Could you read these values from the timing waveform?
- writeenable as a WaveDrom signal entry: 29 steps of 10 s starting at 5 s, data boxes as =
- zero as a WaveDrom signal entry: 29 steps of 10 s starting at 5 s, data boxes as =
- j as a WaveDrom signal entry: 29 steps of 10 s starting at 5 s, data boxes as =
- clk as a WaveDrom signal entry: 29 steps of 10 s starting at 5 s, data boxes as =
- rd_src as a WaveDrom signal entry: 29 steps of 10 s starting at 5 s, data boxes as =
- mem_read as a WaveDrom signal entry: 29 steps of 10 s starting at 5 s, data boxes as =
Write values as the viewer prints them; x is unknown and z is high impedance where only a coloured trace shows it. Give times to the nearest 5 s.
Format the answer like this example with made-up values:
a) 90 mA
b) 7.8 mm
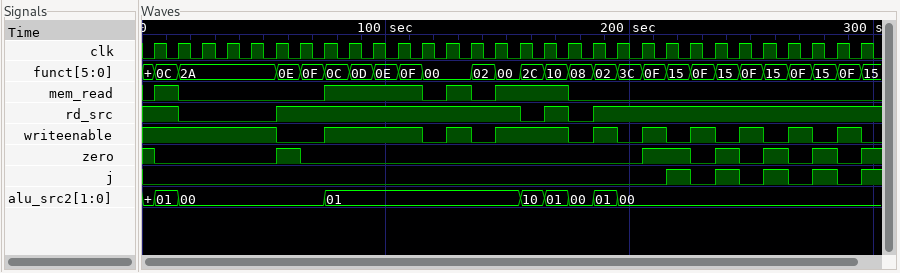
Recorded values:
a) {name: 'writeenable', wave: '1....0.1...0101..010101010101'}
b) {name: 'zero', wave: '0....10.............1.0101010'}
c) {name: 'j', wave: '0....................10101010'}
d) {name: 'clk', wave: 'p............................'}
e) {name: 'rd_src', wave: '10...1.........0101..........'}
f) {name: 'mem_read', wave: '10.....1...0101..0...........'}
